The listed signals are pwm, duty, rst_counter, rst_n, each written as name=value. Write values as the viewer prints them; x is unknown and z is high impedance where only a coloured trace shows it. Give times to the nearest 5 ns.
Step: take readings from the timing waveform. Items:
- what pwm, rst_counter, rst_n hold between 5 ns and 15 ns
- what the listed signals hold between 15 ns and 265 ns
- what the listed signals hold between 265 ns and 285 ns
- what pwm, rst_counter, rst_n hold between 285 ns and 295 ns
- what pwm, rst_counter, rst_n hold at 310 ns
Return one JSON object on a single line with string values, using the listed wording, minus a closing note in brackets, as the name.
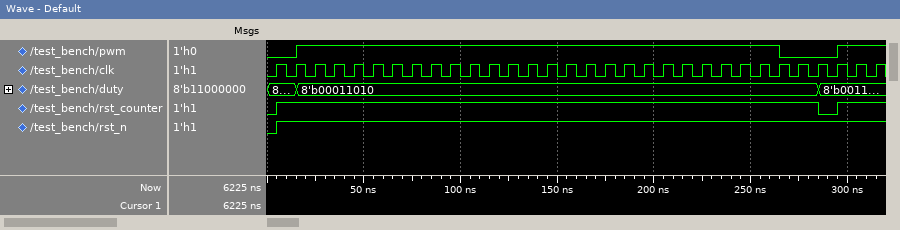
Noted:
{"what pwm, rst_counter, rst_n hold between 5 ns and 15 ns": "pwm=0, rst_counter=1, rst_n=1", "what the listed signals hold between 15 ns and 265 ns": "pwm=1, duty=8'b00011010, rst_counter=1, rst_n=1", "what the listed signals hold between 265 ns and 285 ns": "pwm=0, duty=8'b00011010, rst_counter=1, rst_n=1", "what pwm, rst_counter, rst_n hold between 285 ns and 295 ns": "pwm=0, rst_counter=0, rst_n=1", "what pwm, rst_counter, rst_n hold at 310 ns": "pwm=1, rst_counter=1, rst_n=1"}
